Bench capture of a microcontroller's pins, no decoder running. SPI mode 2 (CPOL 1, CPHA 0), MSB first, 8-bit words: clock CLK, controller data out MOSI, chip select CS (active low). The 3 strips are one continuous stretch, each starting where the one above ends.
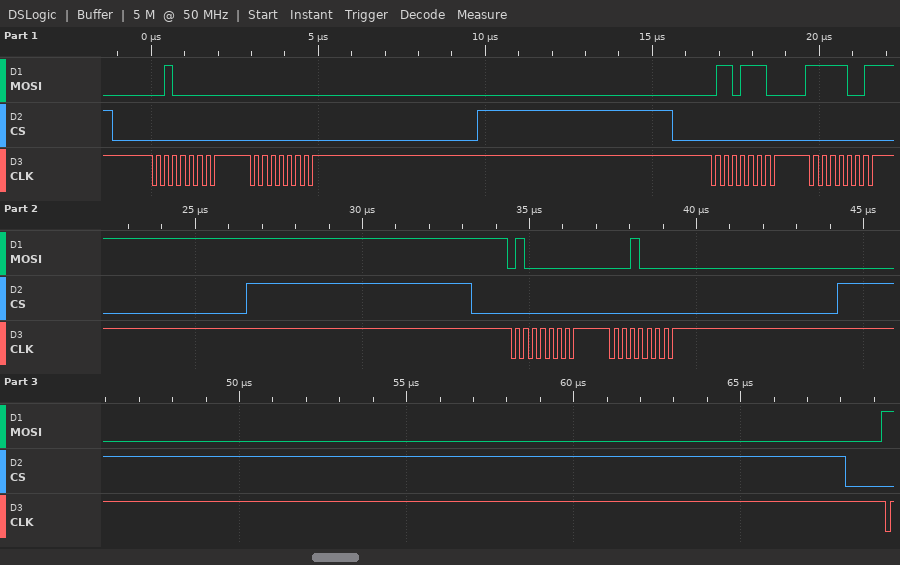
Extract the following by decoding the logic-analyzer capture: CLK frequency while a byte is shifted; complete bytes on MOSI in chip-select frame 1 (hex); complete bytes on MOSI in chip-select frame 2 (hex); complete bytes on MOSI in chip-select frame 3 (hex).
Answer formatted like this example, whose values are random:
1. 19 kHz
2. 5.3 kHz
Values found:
1. 4 MHz
2. 20 00
3. 6E F9
4. 40 10
